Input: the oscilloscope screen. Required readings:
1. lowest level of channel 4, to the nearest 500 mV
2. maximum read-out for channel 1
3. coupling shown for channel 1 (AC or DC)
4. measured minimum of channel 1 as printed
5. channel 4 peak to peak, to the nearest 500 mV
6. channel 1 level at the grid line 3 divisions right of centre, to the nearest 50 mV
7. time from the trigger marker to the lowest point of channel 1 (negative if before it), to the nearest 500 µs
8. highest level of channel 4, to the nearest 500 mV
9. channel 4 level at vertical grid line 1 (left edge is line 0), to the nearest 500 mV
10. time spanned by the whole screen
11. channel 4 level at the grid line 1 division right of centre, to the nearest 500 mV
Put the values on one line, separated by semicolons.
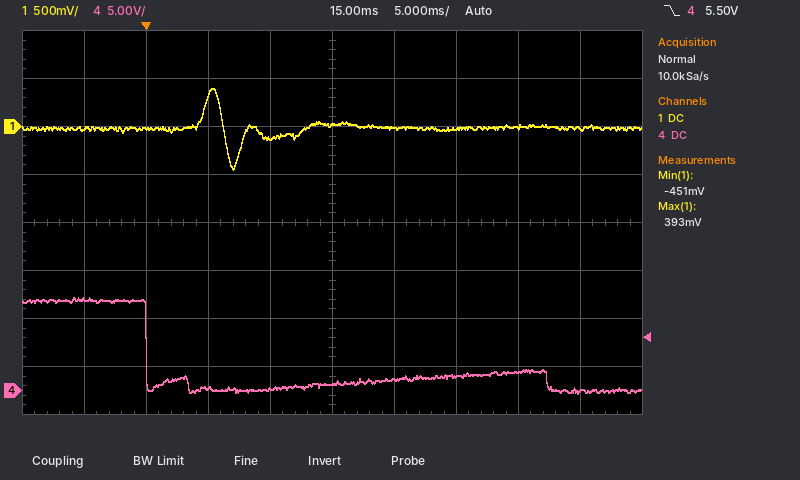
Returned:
-500 mV; 393 mV; DC; -451 mV; 10.0 V; 0 mV; +7.0 ms; 9.5 V; 9.5 V; 50 ms; 1.0 V
